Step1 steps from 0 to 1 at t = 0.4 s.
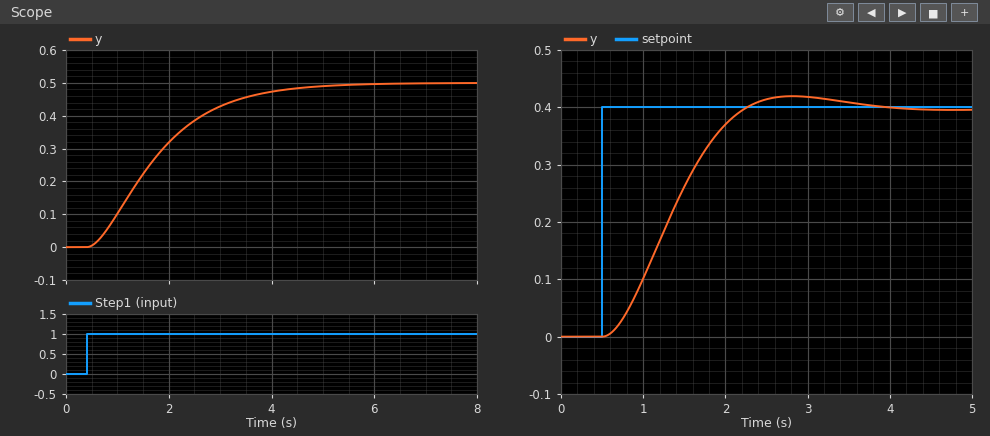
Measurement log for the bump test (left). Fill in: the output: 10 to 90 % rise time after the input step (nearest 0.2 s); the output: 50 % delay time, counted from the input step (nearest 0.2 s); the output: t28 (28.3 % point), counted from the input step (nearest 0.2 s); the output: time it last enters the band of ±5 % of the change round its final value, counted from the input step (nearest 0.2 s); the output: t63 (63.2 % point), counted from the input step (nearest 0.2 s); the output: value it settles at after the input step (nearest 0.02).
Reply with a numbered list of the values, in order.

1. 2.6 s
2. 1.2 s
3. 0.8 s
4. 3.6 s
5. 1.6 s
6. 0.50
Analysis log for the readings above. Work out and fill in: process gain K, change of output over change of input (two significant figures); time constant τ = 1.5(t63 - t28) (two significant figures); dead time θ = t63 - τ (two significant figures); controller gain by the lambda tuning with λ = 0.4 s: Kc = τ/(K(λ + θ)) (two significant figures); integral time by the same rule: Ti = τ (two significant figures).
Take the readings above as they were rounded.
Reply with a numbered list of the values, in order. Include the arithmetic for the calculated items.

1. (0.5 - 0) / 1 = 0.50
2. 1.5 × (1.6 - 0.8) = 1.2 s
3. 1.6 - 1.2 = 0.40 s
4. 1.2 / (0.5 × (0.4 + 0.4)) = 3.0
5. 1.2 s
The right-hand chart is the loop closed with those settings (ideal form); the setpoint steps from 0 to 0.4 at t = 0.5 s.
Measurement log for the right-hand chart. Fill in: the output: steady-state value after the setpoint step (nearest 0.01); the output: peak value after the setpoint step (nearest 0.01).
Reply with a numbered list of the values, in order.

1. 0.40
2. 0.42
